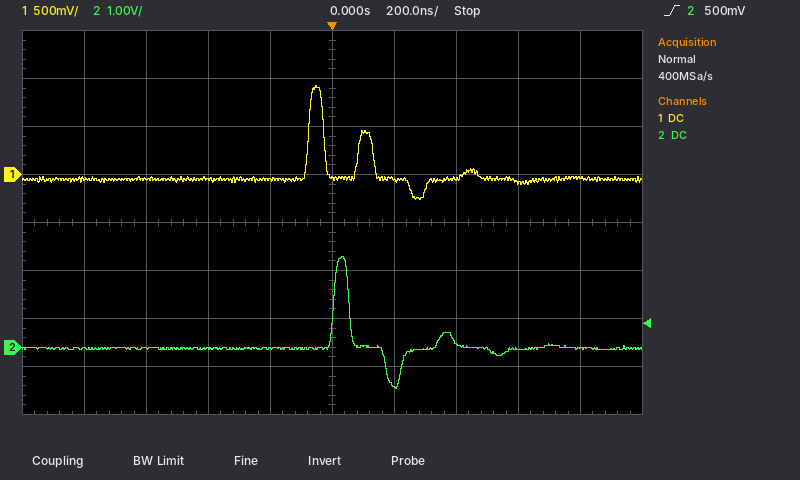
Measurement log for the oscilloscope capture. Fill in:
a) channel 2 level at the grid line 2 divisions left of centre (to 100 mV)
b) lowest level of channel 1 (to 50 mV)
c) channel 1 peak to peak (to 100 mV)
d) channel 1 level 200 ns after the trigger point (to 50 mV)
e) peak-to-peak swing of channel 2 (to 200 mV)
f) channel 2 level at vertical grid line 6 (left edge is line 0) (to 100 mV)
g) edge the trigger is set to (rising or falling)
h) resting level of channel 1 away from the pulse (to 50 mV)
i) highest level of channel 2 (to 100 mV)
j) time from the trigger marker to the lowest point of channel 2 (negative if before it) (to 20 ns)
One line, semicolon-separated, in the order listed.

0.0 V; -250 mV; 1.20 V; -50 mV; 2.8 V; -800 mV; rising; -50 mV; 1.9 V; +200 ns
